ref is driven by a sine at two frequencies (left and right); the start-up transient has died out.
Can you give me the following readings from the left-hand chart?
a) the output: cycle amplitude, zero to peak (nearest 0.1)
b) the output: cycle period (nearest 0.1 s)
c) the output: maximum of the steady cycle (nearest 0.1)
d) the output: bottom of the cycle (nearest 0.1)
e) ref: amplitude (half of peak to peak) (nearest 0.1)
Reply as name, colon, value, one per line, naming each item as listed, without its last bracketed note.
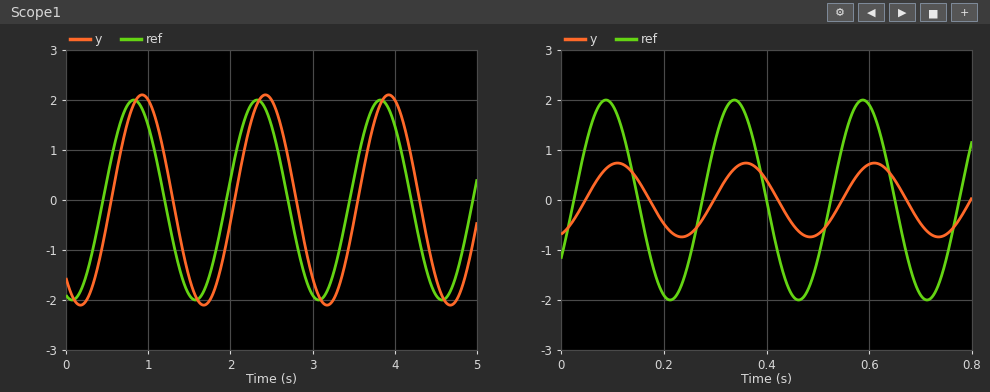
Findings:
the output: cycle amplitude, zero to peak: 2.1
the output: cycle period: 1.5 s
the output: maximum of the steady cycle: 2.1
the output: bottom of the cycle: -2.1
ref: amplitude (half of peak to peak): 2.0
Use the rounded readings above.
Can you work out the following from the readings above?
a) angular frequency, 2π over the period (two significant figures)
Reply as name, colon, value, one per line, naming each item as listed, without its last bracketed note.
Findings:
angular frequency, 2π over the period: 4.2 rad/s
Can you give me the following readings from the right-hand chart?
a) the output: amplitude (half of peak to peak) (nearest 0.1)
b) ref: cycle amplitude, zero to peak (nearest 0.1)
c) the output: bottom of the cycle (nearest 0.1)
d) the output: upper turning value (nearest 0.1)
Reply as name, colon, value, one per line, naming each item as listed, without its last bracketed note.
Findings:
the output: amplitude (half of peak to peak): 0.7
ref: cycle amplitude, zero to peak: 2.0
the output: bottom of the cycle: -0.7
the output: upper turning value: 0.7
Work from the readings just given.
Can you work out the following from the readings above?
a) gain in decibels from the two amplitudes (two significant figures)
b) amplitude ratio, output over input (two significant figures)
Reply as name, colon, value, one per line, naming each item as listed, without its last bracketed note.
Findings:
gain in decibels from the two amplitudes: -9.1 dB
amplitude ratio, output over input: 0.35
